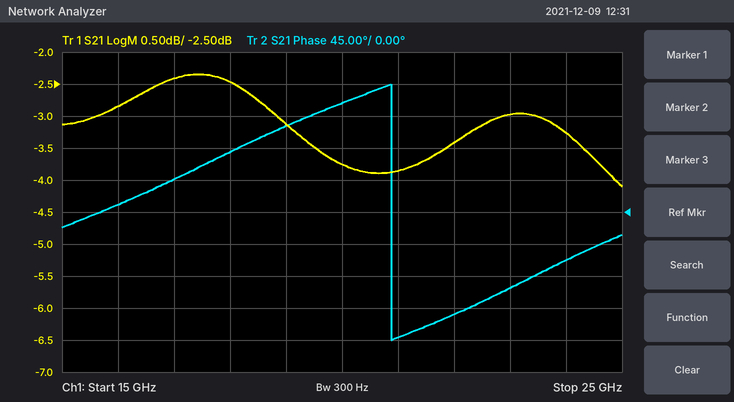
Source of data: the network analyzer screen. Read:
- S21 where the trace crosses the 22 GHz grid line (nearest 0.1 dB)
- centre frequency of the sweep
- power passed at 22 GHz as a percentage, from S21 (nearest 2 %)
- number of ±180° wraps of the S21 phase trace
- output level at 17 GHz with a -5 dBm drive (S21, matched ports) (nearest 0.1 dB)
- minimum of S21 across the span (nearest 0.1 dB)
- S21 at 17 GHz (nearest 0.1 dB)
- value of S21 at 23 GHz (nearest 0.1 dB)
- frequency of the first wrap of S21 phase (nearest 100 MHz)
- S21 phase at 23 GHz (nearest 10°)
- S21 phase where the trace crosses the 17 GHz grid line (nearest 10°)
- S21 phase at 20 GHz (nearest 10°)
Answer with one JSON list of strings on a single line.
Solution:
["-3.4 dB", "20 GHz", "46 %", "1", "-7.4 dBm", "-4.1 dB", "-2.4 dB", "-3.0 dB", "20.9 GHz", "-110°", "50°", "150°"]
